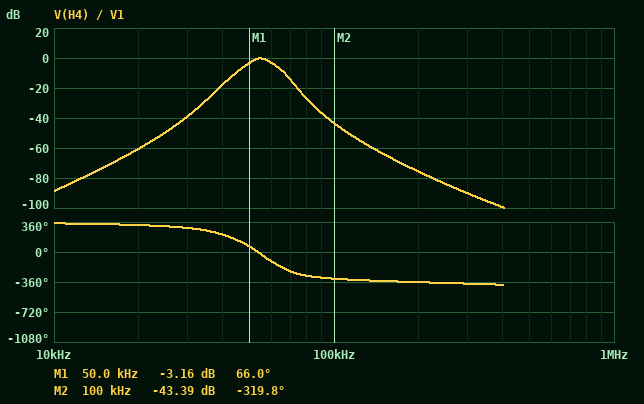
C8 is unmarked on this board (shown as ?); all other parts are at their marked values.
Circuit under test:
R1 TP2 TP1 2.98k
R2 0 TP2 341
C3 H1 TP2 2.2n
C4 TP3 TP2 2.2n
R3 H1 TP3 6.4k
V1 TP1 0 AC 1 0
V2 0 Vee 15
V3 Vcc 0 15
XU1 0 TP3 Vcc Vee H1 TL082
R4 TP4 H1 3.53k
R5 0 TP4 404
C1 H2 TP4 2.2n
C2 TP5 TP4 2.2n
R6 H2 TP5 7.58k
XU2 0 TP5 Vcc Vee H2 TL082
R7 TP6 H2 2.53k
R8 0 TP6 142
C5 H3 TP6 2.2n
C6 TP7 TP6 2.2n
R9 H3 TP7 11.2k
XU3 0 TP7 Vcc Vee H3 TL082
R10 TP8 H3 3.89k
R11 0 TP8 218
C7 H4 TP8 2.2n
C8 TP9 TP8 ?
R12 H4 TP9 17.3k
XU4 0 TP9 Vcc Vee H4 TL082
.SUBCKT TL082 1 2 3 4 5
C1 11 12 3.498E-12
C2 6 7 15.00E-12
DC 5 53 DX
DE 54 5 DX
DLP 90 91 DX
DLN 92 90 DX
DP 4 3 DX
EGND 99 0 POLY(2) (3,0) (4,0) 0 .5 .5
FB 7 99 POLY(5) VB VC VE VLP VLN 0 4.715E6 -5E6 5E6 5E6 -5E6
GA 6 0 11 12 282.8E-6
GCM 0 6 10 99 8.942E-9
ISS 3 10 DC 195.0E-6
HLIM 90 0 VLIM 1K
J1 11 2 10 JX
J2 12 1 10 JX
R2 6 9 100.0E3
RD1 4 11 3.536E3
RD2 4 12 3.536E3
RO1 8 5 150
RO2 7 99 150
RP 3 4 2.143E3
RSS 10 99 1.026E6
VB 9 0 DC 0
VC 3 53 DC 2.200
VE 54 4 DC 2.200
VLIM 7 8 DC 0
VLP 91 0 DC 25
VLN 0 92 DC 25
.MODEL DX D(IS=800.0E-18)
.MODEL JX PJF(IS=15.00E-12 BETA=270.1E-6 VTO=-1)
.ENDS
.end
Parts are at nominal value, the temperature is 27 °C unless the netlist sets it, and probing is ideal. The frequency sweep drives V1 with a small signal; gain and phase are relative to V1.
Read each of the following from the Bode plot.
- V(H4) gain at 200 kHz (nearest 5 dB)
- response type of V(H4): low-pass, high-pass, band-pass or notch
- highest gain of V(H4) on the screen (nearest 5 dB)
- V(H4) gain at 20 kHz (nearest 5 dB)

-75 dB
band-pass
0 dB
-60 dB
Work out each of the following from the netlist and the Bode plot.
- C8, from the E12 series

680 pF
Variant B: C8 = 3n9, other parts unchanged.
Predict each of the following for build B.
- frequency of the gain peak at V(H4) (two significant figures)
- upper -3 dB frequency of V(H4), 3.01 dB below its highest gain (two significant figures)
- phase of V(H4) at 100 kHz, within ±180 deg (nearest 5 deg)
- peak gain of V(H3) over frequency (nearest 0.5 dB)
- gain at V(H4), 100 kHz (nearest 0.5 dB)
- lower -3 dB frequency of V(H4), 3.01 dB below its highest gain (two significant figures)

51 kHz
56 kHz
30 deg
5.0 dB
-47.5 dB
43 kHz
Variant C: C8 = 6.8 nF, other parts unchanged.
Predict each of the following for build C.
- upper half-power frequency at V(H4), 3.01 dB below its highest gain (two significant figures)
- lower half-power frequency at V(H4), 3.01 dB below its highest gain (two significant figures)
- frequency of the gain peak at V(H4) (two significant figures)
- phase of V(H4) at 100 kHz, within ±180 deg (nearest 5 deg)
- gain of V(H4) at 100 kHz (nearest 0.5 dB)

56 kHz
44 kHz
52 kHz
30 deg
-47.5 dB
